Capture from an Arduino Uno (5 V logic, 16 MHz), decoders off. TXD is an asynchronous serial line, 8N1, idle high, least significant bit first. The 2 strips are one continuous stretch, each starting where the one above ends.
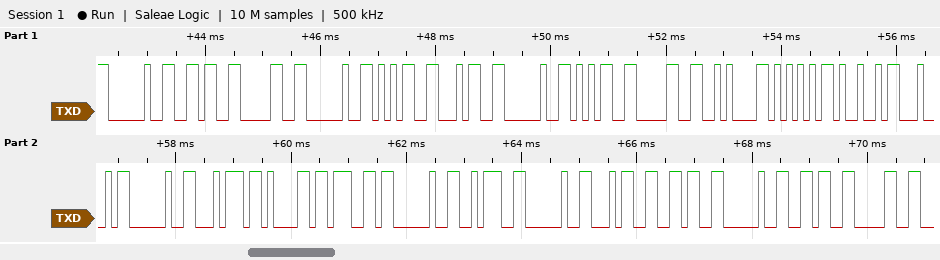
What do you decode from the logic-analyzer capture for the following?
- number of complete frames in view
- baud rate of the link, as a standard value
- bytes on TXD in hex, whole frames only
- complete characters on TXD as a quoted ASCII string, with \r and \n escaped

25
9600 baud
20 36 30 20 35 34 20 35 30 0A 55 49 44 20 74 61 67 20 3A 20 34 36 20 36 30
" 60 54 50\nUID tag : 46 60"
